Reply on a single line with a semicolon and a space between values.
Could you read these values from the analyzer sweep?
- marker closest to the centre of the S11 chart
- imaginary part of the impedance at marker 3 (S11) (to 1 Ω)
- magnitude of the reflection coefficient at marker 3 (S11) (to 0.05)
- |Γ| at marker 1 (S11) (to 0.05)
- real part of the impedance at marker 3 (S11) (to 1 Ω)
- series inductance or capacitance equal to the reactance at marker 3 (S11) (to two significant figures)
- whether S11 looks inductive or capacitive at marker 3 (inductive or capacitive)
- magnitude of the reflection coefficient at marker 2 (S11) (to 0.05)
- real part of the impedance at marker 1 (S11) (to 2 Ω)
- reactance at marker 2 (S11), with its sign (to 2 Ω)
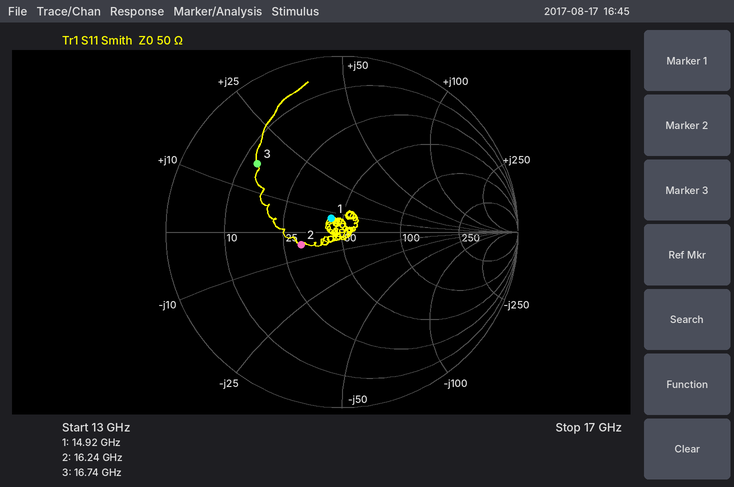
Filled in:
marker 1; +17 Ω; 0.60; 0.10; 13 Ω; 160 pH; inductive; 0.25; 44 Ω; -4 Ω
